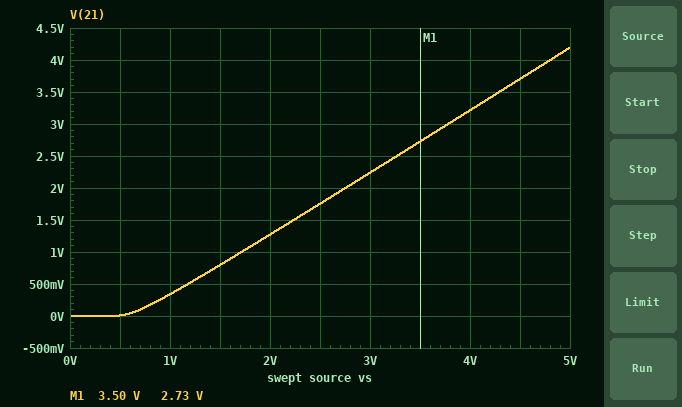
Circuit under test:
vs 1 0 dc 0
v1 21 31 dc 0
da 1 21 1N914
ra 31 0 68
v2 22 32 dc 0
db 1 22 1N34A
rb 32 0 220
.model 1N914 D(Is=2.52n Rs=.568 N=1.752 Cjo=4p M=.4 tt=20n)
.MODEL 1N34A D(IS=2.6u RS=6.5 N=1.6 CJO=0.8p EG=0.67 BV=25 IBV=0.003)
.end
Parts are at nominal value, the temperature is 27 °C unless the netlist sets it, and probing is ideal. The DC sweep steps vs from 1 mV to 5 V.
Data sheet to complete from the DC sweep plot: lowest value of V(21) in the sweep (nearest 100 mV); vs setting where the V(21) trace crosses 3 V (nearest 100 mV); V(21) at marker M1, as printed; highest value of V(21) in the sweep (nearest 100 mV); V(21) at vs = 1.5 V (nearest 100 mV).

0 V
3.8 V
2.73 V
4.2 V
800 mV
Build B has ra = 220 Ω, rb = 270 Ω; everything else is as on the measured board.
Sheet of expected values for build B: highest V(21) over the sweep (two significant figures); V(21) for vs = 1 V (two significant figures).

4.3 V
390 mV
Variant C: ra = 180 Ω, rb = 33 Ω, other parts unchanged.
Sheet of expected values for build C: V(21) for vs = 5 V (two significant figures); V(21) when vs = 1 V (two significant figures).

4.3 V
380 mV
